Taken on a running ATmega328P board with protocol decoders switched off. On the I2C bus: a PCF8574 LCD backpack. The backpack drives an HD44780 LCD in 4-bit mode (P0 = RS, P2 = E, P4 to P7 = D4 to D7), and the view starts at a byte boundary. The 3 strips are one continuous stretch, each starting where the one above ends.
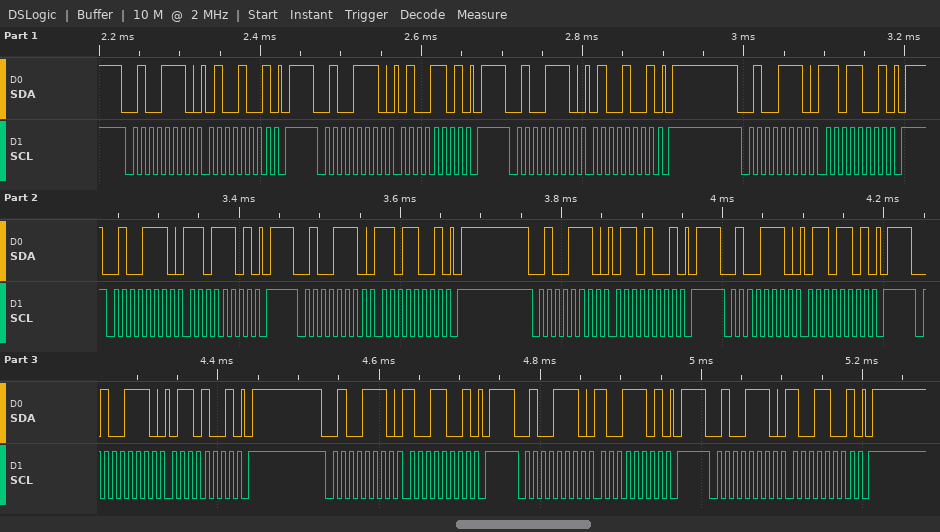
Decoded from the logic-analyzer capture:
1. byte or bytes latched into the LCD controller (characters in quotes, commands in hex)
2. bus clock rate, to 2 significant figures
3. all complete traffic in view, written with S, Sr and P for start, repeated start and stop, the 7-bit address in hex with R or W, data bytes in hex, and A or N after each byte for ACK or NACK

'M' 'i'
100 kHz
S 27W A 49 A P S 27W A 4D A P S 27W A 49 A P S 27W A D9 A P S 27W A DD A P S 27W A D9 A P S 27W A 69 A P S 27W A 6D A P S 27W A 69 A P S 27W A 99 A P S 27W A 9D A P S 27W A 99 A P
